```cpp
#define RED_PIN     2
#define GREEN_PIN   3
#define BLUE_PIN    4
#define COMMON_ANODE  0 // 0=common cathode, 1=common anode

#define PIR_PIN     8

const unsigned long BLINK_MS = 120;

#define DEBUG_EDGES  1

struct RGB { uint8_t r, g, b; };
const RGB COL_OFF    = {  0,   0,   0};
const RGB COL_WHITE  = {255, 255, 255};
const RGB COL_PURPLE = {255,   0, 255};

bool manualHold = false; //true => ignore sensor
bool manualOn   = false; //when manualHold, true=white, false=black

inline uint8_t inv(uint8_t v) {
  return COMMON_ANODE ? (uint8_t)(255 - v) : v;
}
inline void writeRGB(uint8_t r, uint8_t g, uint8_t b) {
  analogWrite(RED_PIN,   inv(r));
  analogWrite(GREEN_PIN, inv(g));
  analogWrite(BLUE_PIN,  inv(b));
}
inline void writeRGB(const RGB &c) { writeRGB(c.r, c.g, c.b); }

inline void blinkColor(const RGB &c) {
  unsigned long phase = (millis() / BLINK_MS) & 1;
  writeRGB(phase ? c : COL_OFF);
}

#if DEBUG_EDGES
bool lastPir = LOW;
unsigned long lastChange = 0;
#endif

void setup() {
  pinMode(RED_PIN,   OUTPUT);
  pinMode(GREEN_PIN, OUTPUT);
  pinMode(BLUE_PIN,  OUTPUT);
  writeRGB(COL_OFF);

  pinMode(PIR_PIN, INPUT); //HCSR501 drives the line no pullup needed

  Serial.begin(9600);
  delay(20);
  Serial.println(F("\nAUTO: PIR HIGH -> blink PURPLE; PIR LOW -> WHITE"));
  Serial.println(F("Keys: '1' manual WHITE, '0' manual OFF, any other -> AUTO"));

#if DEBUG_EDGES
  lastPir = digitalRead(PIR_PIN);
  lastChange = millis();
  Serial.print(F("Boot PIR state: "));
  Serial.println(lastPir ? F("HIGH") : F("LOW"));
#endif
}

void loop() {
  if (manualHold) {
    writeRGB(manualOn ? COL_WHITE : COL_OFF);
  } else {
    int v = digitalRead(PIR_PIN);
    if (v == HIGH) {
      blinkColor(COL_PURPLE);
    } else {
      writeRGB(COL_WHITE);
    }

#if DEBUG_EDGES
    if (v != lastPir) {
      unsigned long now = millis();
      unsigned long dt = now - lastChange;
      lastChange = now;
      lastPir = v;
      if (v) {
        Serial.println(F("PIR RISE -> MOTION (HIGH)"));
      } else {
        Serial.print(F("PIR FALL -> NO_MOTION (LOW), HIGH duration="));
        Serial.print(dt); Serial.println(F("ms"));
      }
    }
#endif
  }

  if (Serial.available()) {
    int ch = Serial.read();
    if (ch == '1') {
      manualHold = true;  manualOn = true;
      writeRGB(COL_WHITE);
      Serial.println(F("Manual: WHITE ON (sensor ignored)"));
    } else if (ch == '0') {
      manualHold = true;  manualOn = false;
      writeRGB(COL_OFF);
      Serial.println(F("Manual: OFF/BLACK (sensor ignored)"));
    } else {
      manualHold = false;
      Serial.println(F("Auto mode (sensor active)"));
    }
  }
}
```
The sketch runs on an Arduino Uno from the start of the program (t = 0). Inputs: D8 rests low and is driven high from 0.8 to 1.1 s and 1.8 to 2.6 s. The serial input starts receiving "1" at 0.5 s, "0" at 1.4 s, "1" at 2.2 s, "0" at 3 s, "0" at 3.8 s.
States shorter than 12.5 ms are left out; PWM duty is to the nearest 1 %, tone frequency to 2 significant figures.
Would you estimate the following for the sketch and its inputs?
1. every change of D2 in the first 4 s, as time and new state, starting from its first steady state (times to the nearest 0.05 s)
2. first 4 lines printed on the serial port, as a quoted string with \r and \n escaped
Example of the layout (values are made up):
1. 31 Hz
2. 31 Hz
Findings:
1. 0 s low; 0.1 s high; 1.4 s low; 2.2 s high; 3 s low
2. "\nAUTO: PIR HIGH -> blink PURPLE; PIR LOW -> WHITE\r\nKeys: '1' manual WHITE, '0' manual OFF, any other -> AUTO\r\nBoot PIR state: LOW\r\n"
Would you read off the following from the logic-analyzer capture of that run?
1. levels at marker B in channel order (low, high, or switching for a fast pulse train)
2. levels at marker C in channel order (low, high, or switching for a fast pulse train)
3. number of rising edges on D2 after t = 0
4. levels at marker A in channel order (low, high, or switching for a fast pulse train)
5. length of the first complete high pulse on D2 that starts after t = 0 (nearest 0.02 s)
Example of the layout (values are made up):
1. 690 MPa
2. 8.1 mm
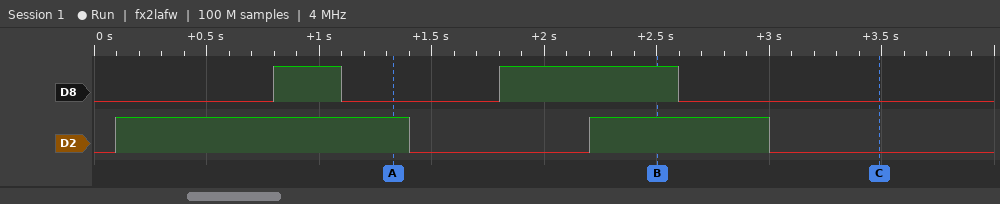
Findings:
1. D8 high, D2 high
2. D8 low, D2 low
3. 2
4. D8 low, D2 high
5. 1.30 s
